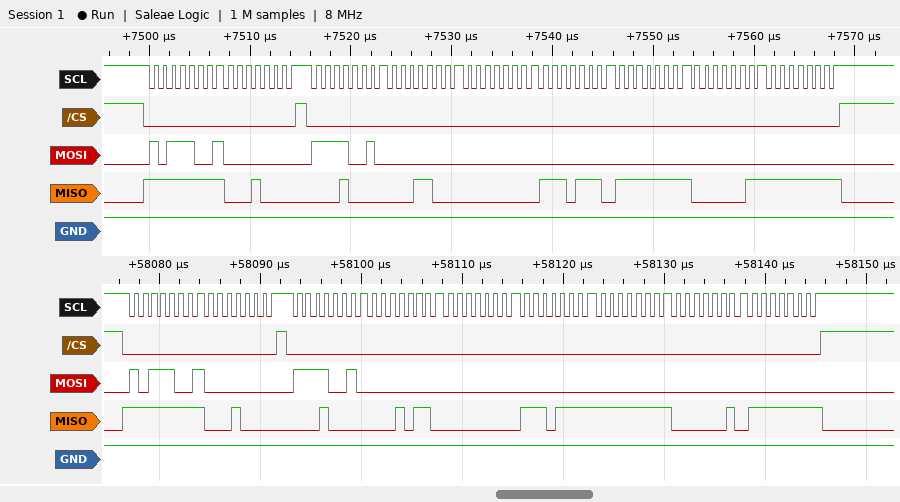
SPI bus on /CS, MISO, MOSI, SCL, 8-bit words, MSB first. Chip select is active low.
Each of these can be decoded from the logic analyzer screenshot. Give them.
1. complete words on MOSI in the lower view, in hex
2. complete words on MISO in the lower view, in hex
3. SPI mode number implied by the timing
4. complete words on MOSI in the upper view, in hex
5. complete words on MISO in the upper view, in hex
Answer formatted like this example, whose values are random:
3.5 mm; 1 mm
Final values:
B9, 00, F2, 00, 00, 00, 00, 00, 00; FF, 10, 10, 16, 00, EF, FF, 02, FF; 3; B9, 00, F2, 00, 00, 00, 00, 00, 00; FF, 10, 10, 18, 00, EE, FF, 03, FF
